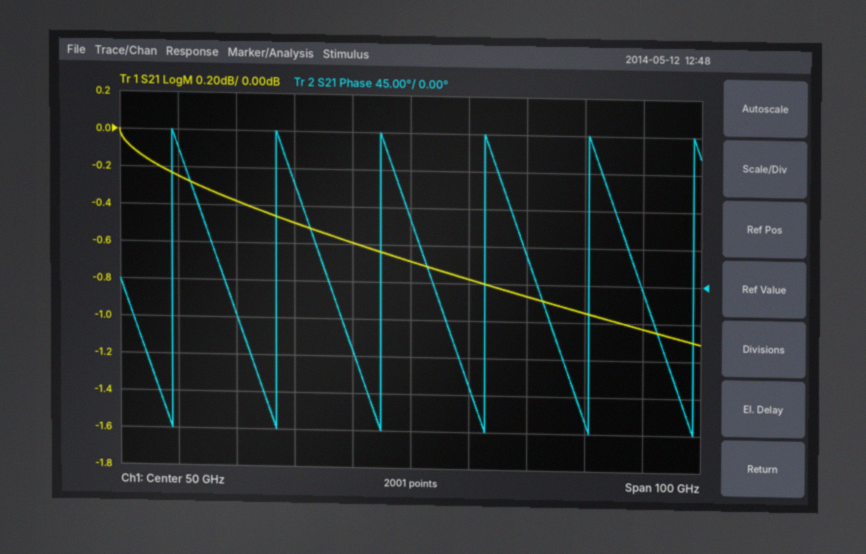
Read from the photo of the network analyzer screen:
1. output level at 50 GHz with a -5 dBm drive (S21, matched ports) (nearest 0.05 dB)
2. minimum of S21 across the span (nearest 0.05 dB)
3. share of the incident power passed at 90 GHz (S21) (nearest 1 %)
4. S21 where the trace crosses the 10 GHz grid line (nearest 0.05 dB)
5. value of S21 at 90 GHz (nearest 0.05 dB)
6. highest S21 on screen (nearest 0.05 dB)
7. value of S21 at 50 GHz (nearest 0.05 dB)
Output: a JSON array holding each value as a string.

["-5.70 dBm", "-1.10 dB", "79 %", "-0.25 dB", "-1.05 dB", "0.00 dB", "-0.70 dB"]
